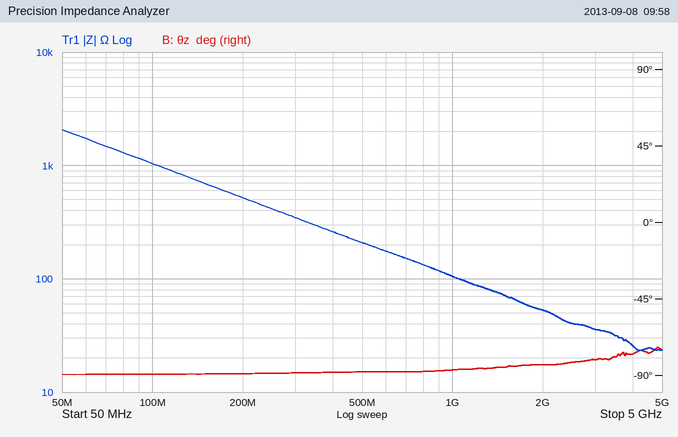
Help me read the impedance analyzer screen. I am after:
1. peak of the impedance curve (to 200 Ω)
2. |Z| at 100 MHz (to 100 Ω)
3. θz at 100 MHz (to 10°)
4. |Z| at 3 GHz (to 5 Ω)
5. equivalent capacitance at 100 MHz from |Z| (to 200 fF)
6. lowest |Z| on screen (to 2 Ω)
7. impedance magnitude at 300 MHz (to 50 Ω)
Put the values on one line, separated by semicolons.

2.0 kΩ; 1.0 kΩ; -90°; 35 Ω; 1.6 pF; 24 Ω; 350 Ω
